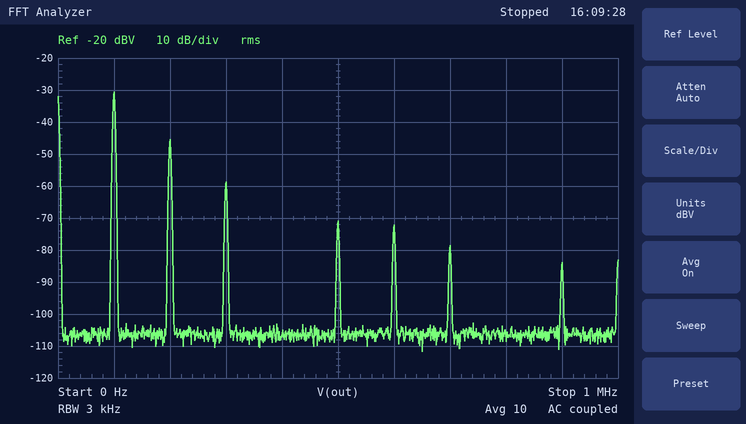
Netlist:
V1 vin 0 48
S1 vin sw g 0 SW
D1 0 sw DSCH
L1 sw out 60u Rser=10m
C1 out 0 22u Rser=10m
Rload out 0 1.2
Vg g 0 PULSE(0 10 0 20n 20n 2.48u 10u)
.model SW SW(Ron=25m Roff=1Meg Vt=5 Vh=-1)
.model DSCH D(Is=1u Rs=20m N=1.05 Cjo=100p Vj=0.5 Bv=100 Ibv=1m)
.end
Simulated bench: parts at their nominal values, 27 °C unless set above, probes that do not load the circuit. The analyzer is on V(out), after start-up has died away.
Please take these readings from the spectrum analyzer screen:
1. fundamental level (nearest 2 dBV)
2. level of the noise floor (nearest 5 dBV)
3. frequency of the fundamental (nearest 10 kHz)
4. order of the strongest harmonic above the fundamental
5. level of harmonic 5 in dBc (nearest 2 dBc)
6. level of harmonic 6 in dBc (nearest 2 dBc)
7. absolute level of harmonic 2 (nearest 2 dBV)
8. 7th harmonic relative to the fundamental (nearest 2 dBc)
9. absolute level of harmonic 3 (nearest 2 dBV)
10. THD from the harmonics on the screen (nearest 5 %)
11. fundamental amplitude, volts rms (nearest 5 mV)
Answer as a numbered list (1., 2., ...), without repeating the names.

1. -30 dBV
2. -105 dBV
3. 100 kHz
4. 2
5. -40 dBc
6. -42 dBc
7. -46 dBV
8. -48 dBc
9. -58 dBV
10. 20 %
11. 30 mV
